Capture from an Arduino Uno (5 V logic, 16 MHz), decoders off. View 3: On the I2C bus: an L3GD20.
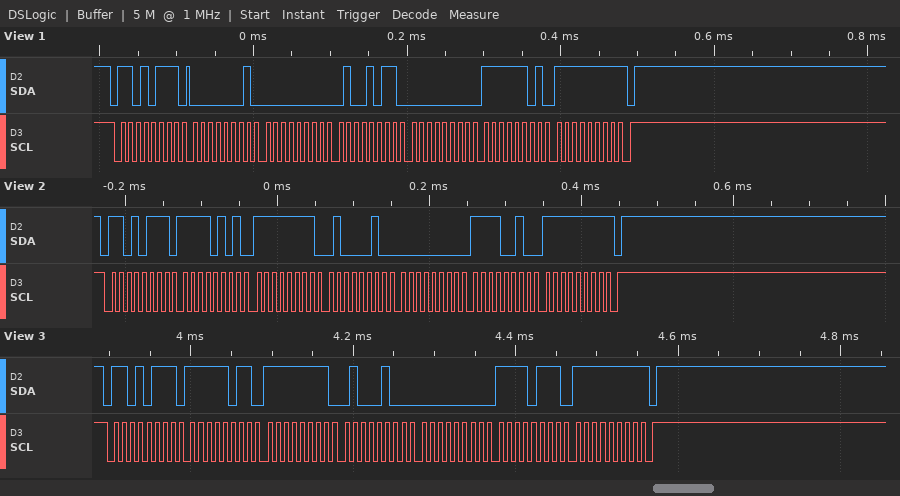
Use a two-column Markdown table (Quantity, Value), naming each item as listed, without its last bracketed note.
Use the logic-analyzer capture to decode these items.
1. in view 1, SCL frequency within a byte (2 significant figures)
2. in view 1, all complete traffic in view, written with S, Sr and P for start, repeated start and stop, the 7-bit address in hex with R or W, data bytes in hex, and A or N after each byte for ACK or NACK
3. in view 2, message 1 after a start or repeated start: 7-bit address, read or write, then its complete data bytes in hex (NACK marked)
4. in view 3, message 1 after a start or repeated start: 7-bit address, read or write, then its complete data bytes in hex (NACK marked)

| Quantity | Value |
|---|---|
| in view 1, SCL frequency within a byte | 100 kHz |
| in view 1, all complete traffic in view, written with S, Sr and P for start, repeated start and stop, the 7-bit address in hex with R or W, data bytes in hex, and A or N after each byte for ACK or NACK | S 6BR A 01 A 00 A 4B A 00 A FD A FF N P |
| in view 2, message 1 after a start or repeated start: 7-bit address, read or write, then its complete data bytes in hex | 0x6B read: F5 FF 42 00 F2 FF NACK |
| in view 3, message 1 after a start or repeated start: 7-bit address, read or write, then its complete data bytes in hex | 0x6B read: FB FF 44 00 F7 FF NACK |
